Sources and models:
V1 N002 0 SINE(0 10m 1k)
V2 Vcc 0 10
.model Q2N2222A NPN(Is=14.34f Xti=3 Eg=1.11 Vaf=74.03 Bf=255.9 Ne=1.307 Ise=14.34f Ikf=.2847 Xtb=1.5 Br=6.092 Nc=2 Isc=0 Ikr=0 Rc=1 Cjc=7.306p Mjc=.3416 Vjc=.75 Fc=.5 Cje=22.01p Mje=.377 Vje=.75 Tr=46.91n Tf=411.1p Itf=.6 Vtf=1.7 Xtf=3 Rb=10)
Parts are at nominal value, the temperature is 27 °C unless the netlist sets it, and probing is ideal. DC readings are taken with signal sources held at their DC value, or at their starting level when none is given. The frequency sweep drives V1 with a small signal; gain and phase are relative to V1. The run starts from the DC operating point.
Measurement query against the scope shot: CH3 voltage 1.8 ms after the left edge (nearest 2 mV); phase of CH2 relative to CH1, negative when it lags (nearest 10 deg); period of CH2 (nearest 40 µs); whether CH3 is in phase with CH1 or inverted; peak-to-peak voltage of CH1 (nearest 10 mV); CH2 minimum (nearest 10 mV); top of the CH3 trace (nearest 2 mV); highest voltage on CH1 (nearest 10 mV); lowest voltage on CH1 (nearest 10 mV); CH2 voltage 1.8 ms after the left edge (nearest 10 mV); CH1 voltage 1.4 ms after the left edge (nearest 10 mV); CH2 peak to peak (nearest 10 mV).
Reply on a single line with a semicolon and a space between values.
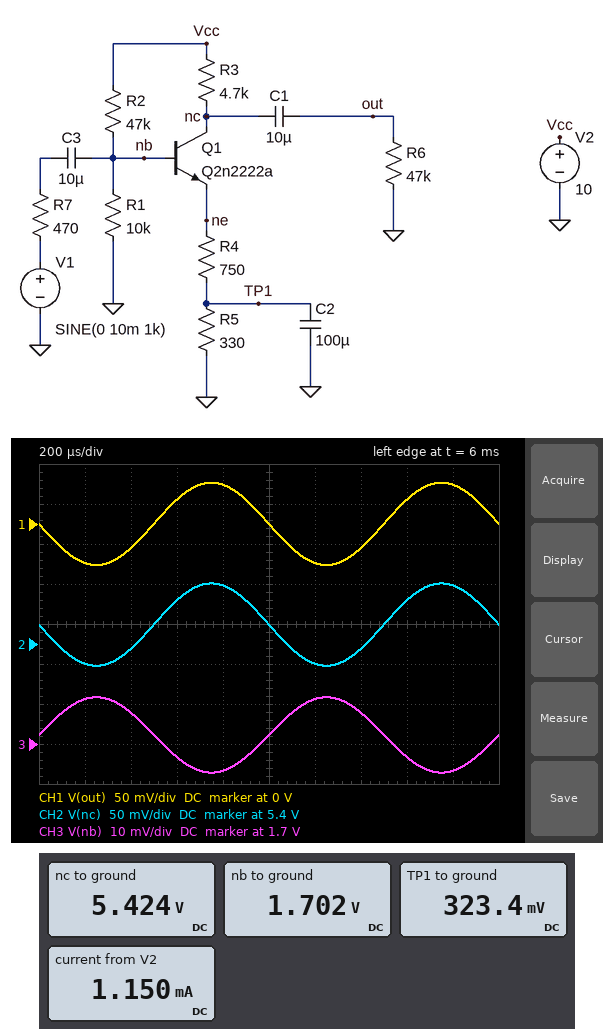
1.694 V; 0 deg; 1.00 ms; inverted; 100 mV; 5.37 V; 1.712 V; 50 mV; -50 mV; 5.47 V; -30 mV; 100 mV
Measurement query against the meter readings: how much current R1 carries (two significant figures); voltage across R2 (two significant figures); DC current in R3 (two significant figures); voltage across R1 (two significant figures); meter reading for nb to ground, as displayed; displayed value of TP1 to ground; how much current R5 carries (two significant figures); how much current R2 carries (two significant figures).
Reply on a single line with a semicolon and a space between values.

170 µA; 8.3 V; 970 µA; 1.7 V; 1.702 V; 323.4 mV; 980 µA; 180 µA
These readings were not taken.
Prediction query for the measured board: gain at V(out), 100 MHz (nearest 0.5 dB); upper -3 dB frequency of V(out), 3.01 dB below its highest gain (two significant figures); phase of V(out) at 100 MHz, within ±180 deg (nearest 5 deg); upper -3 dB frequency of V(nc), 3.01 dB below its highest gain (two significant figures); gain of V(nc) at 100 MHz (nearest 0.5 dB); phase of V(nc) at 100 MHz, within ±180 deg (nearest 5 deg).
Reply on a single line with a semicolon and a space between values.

-3.0 dB; 5.5 MHz; 15 deg; 5.5 MHz; -3.0 dB; 15 deg
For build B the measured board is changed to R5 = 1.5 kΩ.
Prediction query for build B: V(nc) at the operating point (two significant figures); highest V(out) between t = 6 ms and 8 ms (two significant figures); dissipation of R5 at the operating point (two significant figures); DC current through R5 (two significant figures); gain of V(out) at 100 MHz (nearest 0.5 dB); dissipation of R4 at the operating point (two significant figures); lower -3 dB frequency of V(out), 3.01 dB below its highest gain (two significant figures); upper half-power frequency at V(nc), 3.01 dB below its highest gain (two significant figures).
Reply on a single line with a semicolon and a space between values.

7.7 V; 50 mV; 360 µW; 490 µA; -3.0 dB; 180 µW; 3.7 Hz; 6.3 MHz
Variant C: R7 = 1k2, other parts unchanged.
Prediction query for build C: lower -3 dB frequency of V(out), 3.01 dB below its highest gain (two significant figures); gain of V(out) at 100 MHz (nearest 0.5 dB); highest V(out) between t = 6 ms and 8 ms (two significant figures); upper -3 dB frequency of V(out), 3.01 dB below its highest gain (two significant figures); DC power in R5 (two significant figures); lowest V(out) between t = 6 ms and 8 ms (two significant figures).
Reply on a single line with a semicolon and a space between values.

3.8 Hz; -7.5 dB; 47 mV; 3.5 MHz; 320 µW; -47 mV
